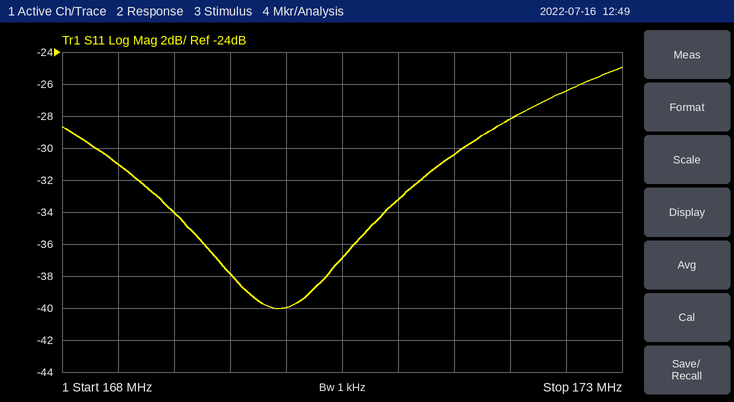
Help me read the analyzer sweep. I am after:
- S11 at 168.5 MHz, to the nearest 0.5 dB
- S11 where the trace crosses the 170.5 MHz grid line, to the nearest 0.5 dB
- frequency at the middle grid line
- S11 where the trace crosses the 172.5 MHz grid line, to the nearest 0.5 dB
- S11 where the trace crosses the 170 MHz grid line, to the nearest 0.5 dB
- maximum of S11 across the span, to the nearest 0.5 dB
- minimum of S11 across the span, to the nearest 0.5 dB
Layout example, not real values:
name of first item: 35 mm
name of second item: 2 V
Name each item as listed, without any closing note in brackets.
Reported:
S11 at 168.5 MHz, to the nearest 0.5 dB: -31.0 dB
S11 where the trace crosses the 170.5 MHz grid line, to the nearest 0.5 dB: -37.0 dB
frequency at the middle grid line: 170.5 MHz
S11 where the trace crosses the 172.5 MHz grid line, to the nearest 0.5 dB: -26.5 dB
S11 where the trace crosses the 170 MHz grid line, to the nearest 0.5 dB: -40.0 dB
maximum of S11 across the span, to the nearest 0.5 dB: -25.0 dB
minimum of S11 across the span, to the nearest 0.5 dB: -40.0 dB
